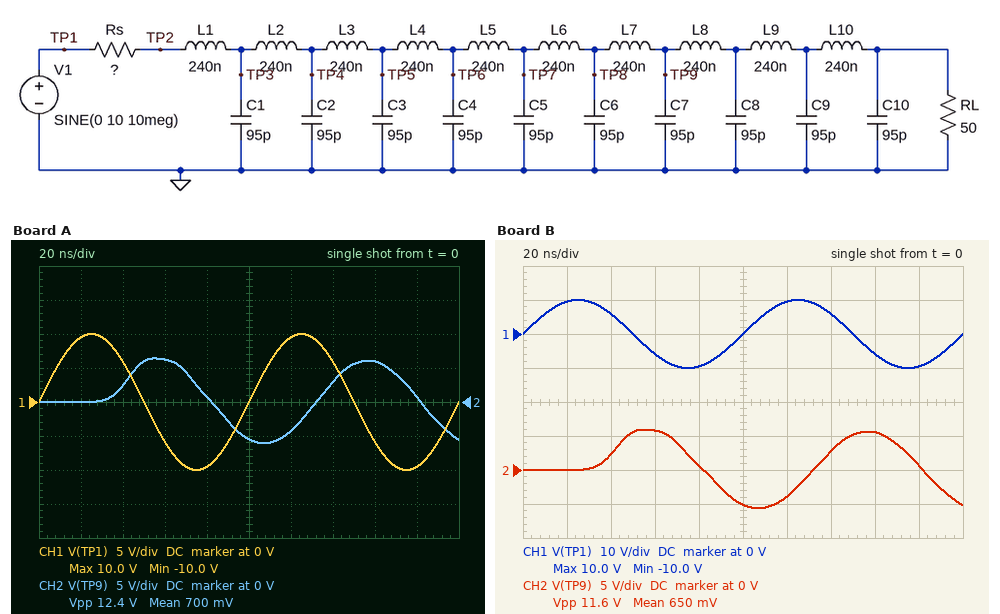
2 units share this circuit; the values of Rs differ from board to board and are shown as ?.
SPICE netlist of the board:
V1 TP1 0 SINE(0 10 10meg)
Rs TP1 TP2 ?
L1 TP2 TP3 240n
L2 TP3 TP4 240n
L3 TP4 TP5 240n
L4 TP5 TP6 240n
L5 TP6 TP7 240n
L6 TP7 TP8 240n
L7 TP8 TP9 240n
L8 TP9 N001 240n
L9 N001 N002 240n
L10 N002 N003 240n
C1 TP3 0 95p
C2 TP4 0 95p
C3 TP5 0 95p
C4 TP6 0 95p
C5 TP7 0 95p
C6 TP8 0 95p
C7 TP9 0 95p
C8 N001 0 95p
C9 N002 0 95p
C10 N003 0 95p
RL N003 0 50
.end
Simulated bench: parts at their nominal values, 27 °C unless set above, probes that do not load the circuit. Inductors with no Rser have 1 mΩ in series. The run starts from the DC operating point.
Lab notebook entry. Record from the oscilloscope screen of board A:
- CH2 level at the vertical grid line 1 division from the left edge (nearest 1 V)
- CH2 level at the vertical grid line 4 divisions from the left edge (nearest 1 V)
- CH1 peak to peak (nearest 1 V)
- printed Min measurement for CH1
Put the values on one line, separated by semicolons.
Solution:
0 V; 1 V; 20 V; -10.0 V
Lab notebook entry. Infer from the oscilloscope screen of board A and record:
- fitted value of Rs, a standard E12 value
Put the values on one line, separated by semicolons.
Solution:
27 Ω
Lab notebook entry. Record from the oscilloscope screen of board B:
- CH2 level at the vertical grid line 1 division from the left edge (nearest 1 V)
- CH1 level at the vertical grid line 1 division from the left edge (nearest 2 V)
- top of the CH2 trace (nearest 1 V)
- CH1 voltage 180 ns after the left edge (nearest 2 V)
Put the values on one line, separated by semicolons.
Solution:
0 V; 10 V; 6 V; -10 V
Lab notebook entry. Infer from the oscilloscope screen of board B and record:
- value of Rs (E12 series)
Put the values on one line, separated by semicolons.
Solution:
33 Ω
